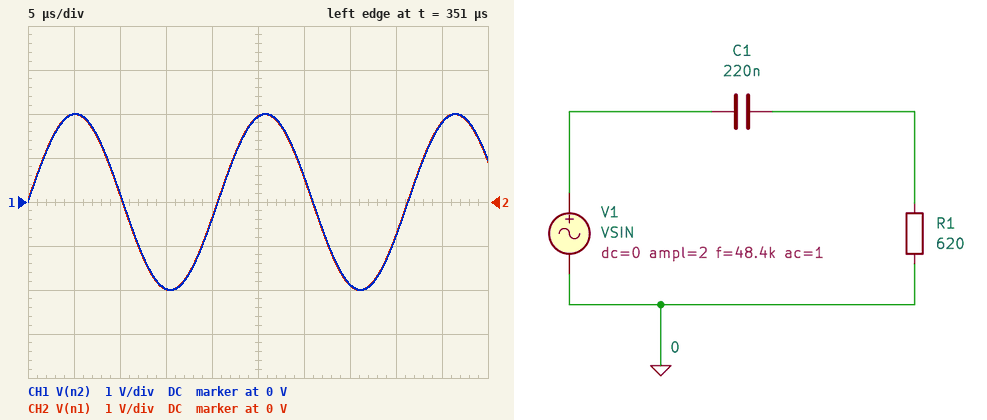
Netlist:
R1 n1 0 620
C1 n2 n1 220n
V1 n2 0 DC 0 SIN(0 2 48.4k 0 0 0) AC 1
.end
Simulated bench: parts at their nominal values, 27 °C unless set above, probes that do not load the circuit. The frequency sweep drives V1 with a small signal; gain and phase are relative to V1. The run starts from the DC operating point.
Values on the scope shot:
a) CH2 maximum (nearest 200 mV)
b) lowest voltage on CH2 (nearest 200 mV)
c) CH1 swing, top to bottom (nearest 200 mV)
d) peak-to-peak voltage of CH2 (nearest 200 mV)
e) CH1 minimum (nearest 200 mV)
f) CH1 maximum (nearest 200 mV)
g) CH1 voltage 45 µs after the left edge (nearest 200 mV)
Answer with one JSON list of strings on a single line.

["2.0 V", "-2.0 V", "4.0 V", "4.0 V", "-2.0 V", "2.0 V", "1.8 V"]
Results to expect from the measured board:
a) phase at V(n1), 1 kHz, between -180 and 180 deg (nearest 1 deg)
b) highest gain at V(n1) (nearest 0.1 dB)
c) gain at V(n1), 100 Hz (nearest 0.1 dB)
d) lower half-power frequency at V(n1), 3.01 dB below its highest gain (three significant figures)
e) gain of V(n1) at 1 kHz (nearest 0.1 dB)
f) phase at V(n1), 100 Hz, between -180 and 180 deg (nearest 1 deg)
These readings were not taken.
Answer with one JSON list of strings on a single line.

["49 deg", "0 dB", "-21.4 dB", "1.17 kHz", "-3.7 dB", "85 deg"]
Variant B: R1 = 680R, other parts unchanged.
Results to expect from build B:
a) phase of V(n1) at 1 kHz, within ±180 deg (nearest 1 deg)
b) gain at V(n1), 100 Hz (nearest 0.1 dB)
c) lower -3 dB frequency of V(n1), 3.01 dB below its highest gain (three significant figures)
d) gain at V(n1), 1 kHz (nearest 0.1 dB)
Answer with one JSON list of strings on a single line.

["47 deg", "-20.6 dB", "1.06 kHz", "-3.3 dB"]
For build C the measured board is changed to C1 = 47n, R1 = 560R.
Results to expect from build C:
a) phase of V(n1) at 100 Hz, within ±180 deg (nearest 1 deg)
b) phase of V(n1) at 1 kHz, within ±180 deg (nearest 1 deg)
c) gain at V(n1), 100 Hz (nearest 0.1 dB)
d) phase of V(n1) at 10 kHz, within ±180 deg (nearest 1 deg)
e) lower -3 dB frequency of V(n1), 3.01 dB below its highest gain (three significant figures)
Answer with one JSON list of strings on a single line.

["89 deg", "81 deg", "-35.6 dB", "31 deg", "6.05 kHz"]
